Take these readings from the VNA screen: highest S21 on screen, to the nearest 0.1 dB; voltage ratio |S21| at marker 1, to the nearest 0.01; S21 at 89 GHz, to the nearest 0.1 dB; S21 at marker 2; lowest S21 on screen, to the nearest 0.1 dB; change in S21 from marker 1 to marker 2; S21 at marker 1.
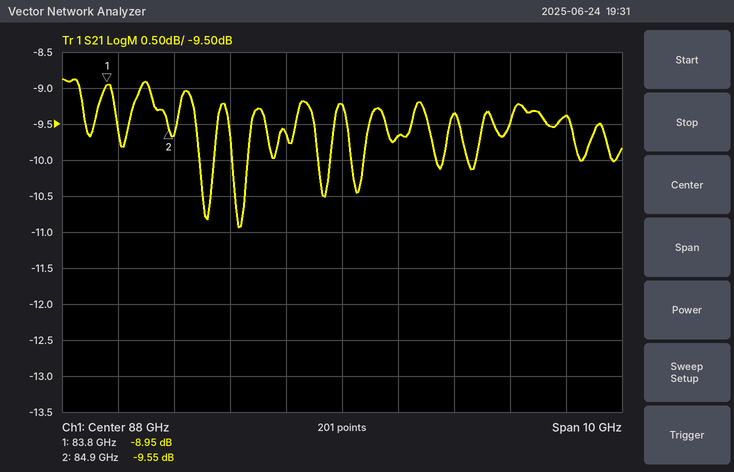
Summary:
-8.9 dB
0.36
-9.7 dB
-9.55 dB
-10.9 dB
-0.60 dB
-8.95 dB
